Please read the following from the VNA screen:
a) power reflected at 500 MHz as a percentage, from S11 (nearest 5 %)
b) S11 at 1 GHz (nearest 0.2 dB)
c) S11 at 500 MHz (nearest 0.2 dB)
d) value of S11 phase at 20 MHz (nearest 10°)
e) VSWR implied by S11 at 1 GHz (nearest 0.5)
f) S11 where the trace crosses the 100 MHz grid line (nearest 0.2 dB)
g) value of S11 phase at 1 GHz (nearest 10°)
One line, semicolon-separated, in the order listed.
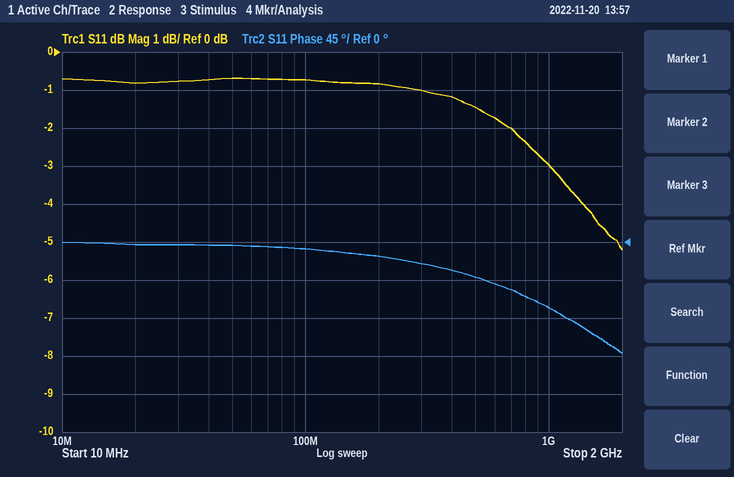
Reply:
70 %; -3.0 dB; -1.4 dB; 0°; 6.0; -0.8 dB; -80°
